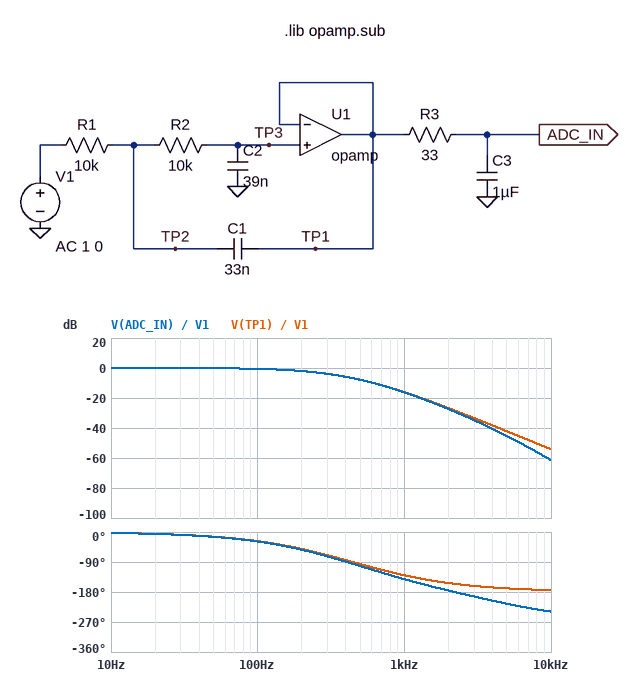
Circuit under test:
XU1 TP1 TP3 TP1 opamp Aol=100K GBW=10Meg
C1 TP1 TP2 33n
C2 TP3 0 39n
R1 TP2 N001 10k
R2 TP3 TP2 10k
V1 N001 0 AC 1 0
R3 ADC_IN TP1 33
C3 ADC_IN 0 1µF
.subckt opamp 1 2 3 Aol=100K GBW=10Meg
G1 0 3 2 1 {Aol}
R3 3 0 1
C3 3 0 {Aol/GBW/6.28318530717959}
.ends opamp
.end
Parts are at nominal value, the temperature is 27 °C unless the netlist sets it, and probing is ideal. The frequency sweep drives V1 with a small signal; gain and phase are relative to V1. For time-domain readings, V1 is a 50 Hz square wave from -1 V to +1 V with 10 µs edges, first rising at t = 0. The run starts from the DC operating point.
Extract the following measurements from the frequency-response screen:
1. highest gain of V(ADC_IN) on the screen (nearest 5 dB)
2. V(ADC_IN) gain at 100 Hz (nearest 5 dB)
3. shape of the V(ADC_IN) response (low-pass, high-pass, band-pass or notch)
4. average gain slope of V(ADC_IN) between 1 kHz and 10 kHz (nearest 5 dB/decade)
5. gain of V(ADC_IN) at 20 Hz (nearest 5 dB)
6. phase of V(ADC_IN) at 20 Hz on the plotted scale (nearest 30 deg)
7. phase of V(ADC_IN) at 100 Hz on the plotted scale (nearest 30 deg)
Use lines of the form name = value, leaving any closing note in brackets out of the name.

highest gain of V(ADC_IN) on the screen = 0 dB
V(ADC_IN) gain at 100 Hz = 0 dB
shape of the V(ADC_IN) response = low-pass
average gain slope of V(ADC_IN) between 1 kHz and 10 kHz = -45 dB/decade
gain of V(ADC_IN) at 20 Hz = 0 dB
phase of V(ADC_IN) at 20 Hz on the plotted scale = 0 deg
phase of V(ADC_IN) at 100 Hz on the plotted scale = -30 deg
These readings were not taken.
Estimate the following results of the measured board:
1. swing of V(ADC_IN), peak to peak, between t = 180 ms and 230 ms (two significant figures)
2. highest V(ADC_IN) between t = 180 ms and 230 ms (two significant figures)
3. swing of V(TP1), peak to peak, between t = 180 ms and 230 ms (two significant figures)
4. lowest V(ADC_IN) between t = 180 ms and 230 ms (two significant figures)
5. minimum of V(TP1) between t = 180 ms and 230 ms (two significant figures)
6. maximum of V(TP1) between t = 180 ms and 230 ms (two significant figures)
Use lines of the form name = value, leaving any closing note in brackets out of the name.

swing of V(ADC_IN), peak to peak, between t = 180 ms and 230 ms = 2.0 V
highest V(ADC_IN) between t = 180 ms and 230 ms = 1.0 V
swing of V(TP1), peak to peak, between t = 180 ms and 230 ms = 2.0 V
lowest V(ADC_IN) between t = 180 ms and 230 ms = -1.0 V
minimum of V(TP1) between t = 180 ms and 230 ms = -1.0 V
maximum of V(TP1) between t = 180 ms and 230 ms = 1.0 V
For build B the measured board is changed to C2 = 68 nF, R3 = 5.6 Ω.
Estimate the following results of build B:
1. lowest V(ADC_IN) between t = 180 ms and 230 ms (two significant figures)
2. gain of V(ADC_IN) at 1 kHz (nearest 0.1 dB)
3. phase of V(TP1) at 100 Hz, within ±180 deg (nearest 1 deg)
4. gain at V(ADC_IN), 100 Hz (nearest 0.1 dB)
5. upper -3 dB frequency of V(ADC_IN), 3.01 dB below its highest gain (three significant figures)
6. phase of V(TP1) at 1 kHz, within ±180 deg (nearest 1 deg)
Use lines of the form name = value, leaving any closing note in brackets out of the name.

lowest V(ADC_IN) between t = 180 ms and 230 ms = -1.0 V
gain of V(ADC_IN) at 1 kHz = -21.3 dB
phase of V(TP1) at 100 Hz, within ±180 deg = -43 deg
gain at V(ADC_IN), 100 Hz = -1.9 dB
upper -3 dB frequency of V(ADC_IN), 3.01 dB below its highest gain = 133 Hz
phase of V(TP1) at 1 kHz, within ±180 deg = -133 deg
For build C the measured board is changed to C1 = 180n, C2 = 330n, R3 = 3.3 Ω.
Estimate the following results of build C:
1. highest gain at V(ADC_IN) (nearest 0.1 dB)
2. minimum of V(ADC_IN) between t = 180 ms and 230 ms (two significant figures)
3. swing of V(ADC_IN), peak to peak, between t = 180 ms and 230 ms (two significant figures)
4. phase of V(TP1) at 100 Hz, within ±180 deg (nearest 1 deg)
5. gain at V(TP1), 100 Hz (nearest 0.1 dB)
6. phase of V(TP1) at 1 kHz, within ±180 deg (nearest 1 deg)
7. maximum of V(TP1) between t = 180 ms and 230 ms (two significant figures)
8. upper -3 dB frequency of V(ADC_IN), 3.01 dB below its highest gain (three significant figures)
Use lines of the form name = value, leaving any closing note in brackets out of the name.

highest gain at V(ADC_IN) = 0 dB
minimum of V(ADC_IN) between t = 180 ms and 230 ms = -660 mV
swing of V(ADC_IN), peak to peak, between t = 180 ms and 230 ms = 1.3 V
phase of V(TP1) at 100 Hz, within ±180 deg = -108 deg
gain at V(TP1), 100 Hz = -12.8 dB
phase of V(TP1) at 1 kHz, within ±180 deg = -170 deg
maximum of V(TP1) between t = 180 ms and 230 ms = 660 mV
upper -3 dB frequency of V(ADC_IN), 3.01 dB below its highest gain = 27.8 Hz
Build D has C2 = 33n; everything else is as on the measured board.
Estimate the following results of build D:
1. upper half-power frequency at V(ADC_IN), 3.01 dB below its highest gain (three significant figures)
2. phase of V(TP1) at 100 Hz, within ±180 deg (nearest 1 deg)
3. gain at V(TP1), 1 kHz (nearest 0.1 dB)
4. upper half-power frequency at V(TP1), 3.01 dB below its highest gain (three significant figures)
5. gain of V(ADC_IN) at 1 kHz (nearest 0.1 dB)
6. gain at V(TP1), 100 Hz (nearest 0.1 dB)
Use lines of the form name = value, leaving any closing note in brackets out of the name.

upper half-power frequency at V(ADC_IN), 3.01 dB below its highest gain = 309 Hz
phase of V(TP1) at 100 Hz, within ±180 deg = -23 deg
gain at V(TP1), 1 kHz = -14.5 dB
upper half-power frequency at V(TP1), 3.01 dB below its highest gain = 310 Hz
gain of V(ADC_IN) at 1 kHz = -14.7 dB
gain at V(TP1), 100 Hz = -0.4 dB
